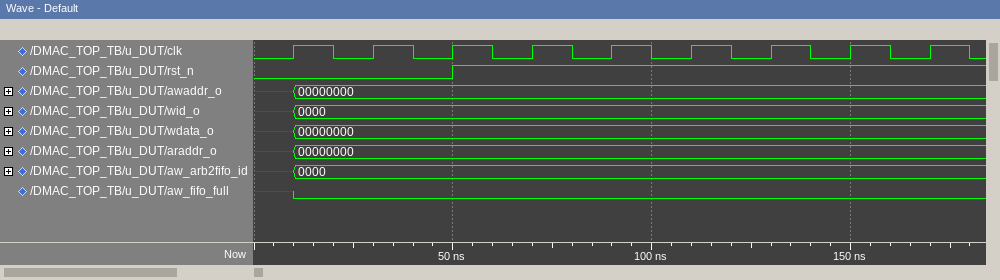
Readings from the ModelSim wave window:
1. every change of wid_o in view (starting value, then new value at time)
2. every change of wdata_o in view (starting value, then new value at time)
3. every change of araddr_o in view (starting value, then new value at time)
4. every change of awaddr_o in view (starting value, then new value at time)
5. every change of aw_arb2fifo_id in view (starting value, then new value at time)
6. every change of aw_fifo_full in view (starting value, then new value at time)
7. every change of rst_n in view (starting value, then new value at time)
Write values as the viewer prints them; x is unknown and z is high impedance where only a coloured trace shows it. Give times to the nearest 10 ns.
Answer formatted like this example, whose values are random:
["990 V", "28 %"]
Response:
["x, 0000 at 10 ns", "x, 00000000 at 10 ns", "x, 00000000 at 10 ns", "x, 00000000 at 10 ns", "x, 0000 at 10 ns", "x, 0 at 10 ns", "0, 1 at 50 ns"]
